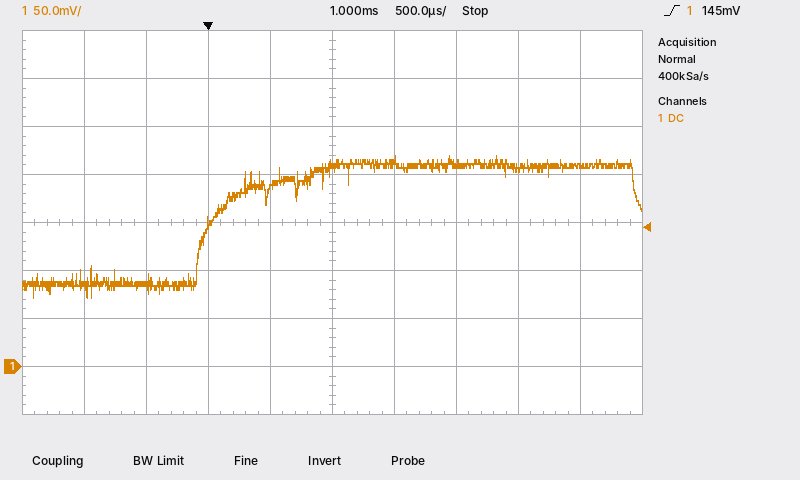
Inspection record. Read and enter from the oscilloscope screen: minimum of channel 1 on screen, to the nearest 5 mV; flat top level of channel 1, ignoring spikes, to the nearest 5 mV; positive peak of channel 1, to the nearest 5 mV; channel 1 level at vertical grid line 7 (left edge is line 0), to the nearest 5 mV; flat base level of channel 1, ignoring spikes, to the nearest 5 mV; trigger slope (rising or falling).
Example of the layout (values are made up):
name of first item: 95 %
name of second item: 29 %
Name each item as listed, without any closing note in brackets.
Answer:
minimum of channel 1 on screen, to the nearest 5 mV: 70 mV
flat top level of channel 1, ignoring spikes, to the nearest 5 mV: 210 mV
positive peak of channel 1, to the nearest 5 mV: 220 mV
channel 1 level at vertical grid line 7 (left edge is line 0), to the nearest 5 mV: 210 mV
flat base level of channel 1, ignoring spikes, to the nearest 5 mV: 85 mV
trigger slope: rising
